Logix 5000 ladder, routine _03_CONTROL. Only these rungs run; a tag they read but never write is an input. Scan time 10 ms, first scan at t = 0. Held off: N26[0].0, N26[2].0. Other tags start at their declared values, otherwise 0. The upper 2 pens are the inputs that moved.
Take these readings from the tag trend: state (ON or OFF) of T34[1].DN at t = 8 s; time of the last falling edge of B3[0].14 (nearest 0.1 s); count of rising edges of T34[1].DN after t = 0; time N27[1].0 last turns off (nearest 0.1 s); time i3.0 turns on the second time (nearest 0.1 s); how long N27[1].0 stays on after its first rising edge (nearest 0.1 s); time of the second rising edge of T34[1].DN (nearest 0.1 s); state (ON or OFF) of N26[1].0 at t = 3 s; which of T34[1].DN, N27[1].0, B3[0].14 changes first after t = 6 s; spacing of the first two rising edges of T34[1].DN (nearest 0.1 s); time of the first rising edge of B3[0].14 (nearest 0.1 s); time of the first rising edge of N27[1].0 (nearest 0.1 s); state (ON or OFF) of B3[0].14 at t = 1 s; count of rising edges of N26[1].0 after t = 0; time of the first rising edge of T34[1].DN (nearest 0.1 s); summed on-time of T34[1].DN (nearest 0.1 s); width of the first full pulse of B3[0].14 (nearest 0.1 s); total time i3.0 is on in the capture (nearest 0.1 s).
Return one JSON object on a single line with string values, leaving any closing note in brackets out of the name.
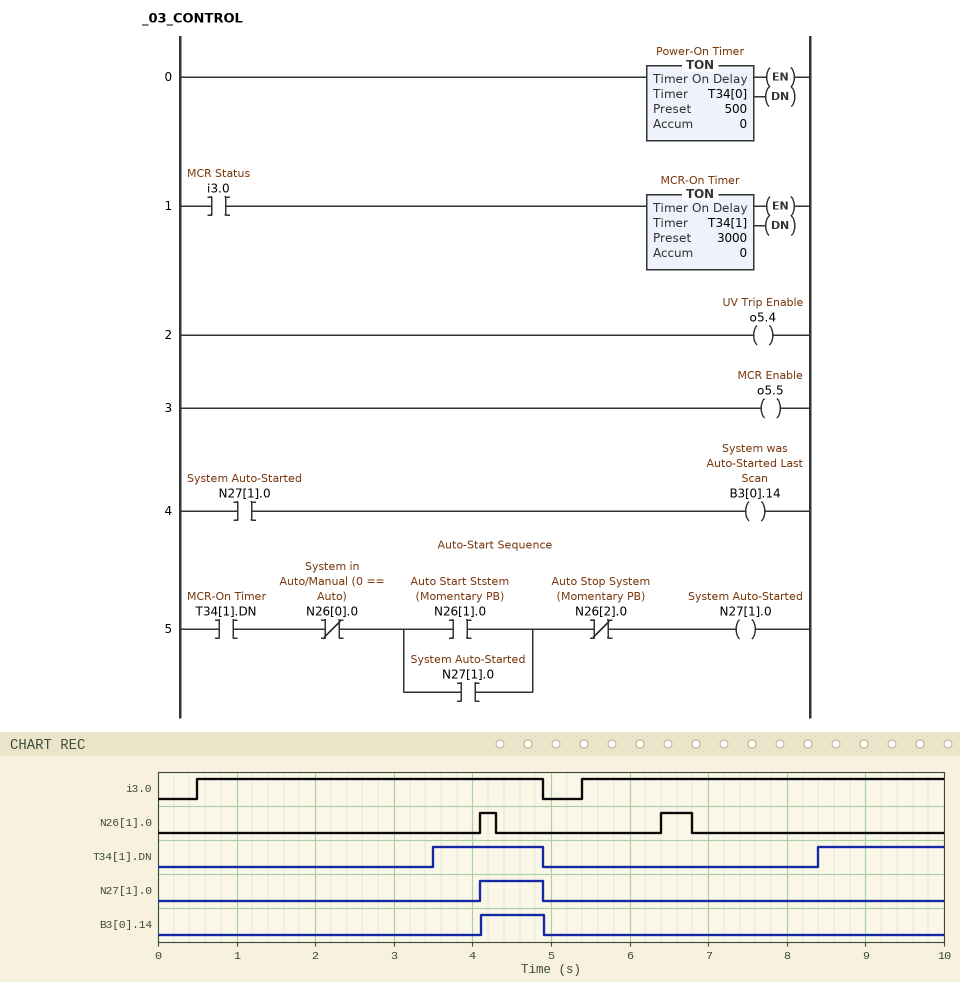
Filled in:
{"state (ON or OFF) of T34[1].DN at t = 8 s": "OFF", "time of the last falling edge of B3[0].14": "4.9 s", "count of rising edges of T34[1].DN after t = 0": "2", "time N27[1].0 last turns off": "4.9 s", "time i3.0 turns on the second time": "5.4 s", "how long N27[1].0 stays on after its first rising edge": "0.8 s", "time of the second rising edge of T34[1].DN": "8.4 s", "state (ON or OFF) of N26[1].0 at t = 3 s": "OFF", "which of T34[1].DN, N27[1].0, B3[0].14 changes first after t = 6 s": "T34[1].DN", "spacing of the first two rising edges of T34[1].DN": "4.9 s", "time of the first rising edge of B3[0].14": "4.1 s", "time of the first rising edge of N27[1].0": "4.1 s", "state (ON or OFF) of B3[0].14 at t = 1 s": "OFF", "count of rising edges of N26[1].0 after t = 0": "2", "time of the first rising edge of T34[1].DN": "3.5 s", "summed on-time of T34[1].DN": "3.0 s", "width of the first full pulse of B3[0].14": "0.8 s", "total time i3.0 is on in the capture": "9.0 s"}
